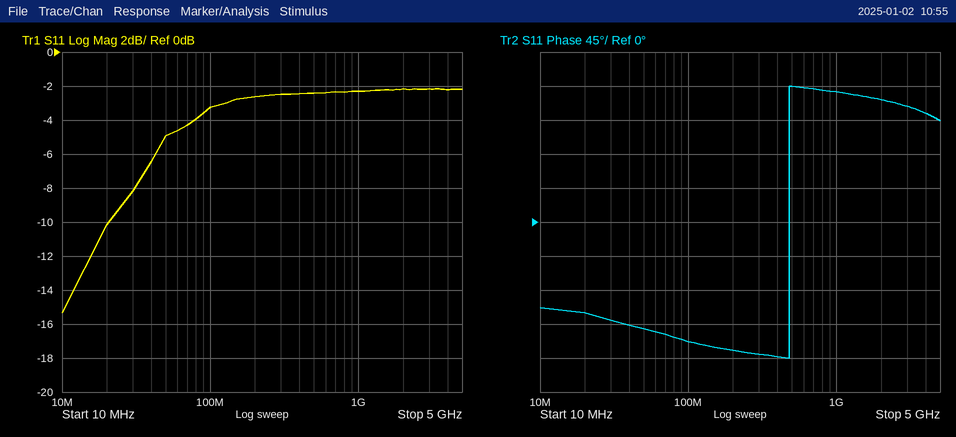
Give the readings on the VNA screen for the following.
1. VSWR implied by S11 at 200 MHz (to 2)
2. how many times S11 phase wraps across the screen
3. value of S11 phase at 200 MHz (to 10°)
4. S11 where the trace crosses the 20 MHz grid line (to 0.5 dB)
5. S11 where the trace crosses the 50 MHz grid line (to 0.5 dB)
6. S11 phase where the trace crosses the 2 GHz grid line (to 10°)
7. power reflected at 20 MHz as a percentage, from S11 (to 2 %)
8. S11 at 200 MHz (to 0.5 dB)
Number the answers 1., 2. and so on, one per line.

1. 6
2. 1
3. -170°
4. -10.0 dB
5. -5.0 dB
6. 160°
7. 10 %
8. -2.5 dB
